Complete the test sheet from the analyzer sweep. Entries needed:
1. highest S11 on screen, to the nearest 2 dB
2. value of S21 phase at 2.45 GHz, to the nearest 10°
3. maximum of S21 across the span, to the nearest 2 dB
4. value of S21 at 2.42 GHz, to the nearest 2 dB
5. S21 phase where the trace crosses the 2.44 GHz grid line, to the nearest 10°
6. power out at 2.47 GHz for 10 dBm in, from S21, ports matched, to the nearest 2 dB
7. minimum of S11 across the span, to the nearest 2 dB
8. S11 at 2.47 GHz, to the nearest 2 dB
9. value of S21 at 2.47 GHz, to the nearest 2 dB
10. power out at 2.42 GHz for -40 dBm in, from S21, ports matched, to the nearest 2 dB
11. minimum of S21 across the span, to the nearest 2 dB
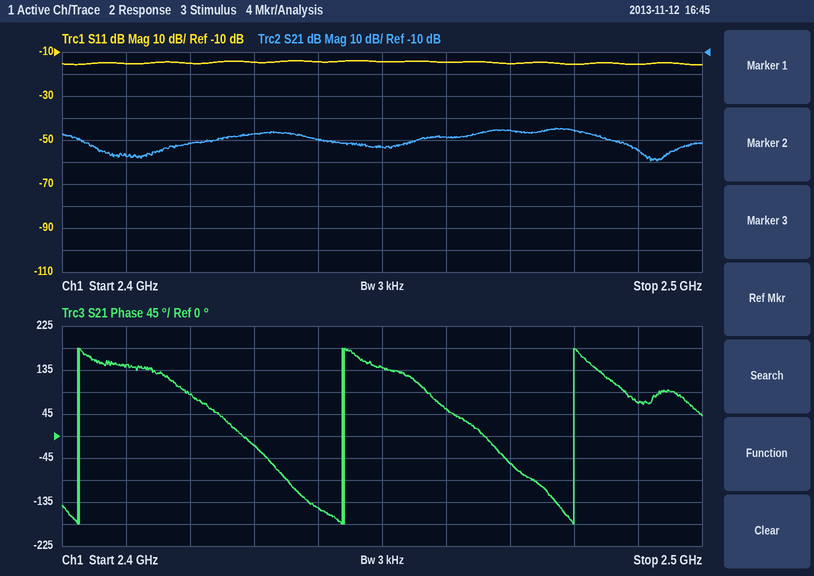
-14 dB
140°
-44 dB
-52 dB
-150°
-36 dBm
-16 dB
-16 dB
-46 dB
-92 dBm
-60 dB
